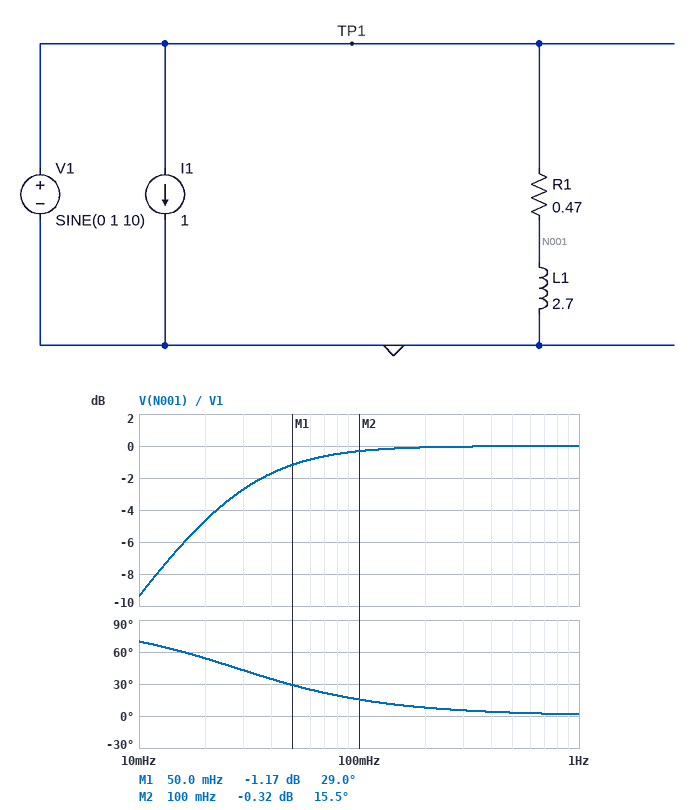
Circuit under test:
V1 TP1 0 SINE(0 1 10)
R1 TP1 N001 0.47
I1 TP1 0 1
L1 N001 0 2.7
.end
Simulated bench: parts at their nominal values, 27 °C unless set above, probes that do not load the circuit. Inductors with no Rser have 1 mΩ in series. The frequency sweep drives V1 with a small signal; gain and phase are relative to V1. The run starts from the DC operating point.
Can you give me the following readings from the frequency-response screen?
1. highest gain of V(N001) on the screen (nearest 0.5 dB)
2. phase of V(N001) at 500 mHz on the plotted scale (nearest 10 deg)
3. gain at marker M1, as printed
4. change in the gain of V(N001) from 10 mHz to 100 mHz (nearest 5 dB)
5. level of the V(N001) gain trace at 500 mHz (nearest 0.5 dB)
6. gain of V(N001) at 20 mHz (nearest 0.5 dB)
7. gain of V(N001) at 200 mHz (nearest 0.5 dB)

0 dB
0 deg
-1.17 dB
10 dB
0 dB
-4.5 dB
0 dB
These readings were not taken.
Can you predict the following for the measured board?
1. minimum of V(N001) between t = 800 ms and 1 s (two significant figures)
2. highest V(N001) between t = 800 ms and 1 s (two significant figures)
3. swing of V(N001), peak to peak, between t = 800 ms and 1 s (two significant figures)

-1.0 V
1.0 V
2.0 V
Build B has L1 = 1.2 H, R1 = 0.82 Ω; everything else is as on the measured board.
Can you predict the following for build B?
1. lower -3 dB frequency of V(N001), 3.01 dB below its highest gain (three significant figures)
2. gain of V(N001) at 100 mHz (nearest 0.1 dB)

109 mHz
-3.4 dB
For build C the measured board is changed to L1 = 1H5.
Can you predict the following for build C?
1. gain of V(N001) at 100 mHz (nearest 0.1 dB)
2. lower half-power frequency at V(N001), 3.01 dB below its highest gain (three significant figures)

-1.0 dB
50.0 mHz
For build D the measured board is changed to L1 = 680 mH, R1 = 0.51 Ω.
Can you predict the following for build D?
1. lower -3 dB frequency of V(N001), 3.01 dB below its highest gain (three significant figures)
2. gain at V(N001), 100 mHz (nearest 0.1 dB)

120 mHz
-3.9 dB
